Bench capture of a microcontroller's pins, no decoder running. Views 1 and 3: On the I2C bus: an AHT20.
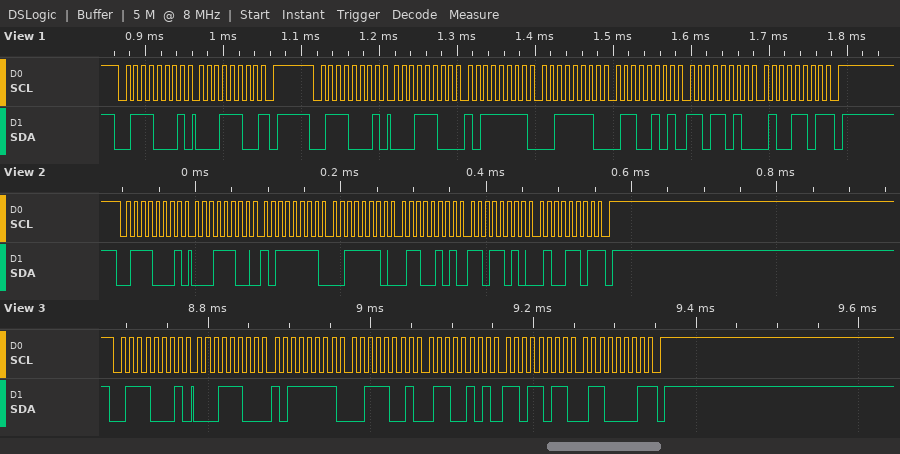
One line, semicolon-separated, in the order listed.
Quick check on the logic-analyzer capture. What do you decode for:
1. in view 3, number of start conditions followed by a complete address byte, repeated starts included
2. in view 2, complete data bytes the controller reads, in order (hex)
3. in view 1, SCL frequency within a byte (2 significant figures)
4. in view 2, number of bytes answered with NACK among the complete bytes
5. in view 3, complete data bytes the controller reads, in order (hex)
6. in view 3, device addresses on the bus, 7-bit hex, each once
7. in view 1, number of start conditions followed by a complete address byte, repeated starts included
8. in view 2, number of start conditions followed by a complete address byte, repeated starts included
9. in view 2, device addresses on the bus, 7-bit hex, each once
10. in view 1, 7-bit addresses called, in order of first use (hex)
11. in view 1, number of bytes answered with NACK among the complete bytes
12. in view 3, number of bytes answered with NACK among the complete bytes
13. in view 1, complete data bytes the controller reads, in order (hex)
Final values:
1; 1C BF 3E 65 DA 4D; 100 kHz; 1; 1C BF 39 65 DB 61; 0x38; 2; 1; 0x38; 0x38; 2; 1; 1C 1C BF 3E 65 DA 4D
